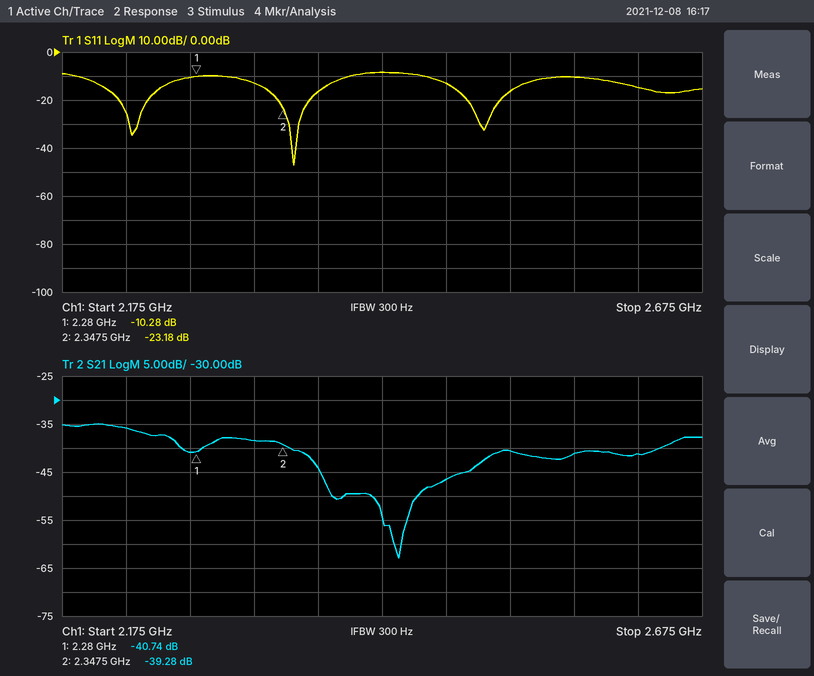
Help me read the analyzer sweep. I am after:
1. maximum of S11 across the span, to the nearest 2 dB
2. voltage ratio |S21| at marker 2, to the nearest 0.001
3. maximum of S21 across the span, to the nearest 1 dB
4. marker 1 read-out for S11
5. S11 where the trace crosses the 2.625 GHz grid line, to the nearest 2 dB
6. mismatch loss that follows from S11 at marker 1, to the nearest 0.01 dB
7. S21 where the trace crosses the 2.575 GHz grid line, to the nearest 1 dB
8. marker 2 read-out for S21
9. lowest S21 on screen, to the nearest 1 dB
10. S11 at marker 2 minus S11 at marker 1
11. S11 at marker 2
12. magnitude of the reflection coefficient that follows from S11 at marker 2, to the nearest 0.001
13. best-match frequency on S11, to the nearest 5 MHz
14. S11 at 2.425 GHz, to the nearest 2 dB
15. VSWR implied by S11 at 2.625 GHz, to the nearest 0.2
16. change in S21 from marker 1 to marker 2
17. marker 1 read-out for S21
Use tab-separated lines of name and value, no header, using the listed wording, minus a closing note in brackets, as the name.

maximum of S11 across the span, to the nearest 2 dB	-8 dB
voltage ratio |S21| at marker 2, to the nearest 0.001	0.011
maximum of S21 across the span, to the nearest 1 dB	-35 dB
marker 1 read-out for S11	-10.28 dB
S11 where the trace crosses the 2.625 GHz grid line, to the nearest 2 dB	-14 dB
mismatch loss that follows from S11 at marker 1, to the nearest 0.01 dB	0.43 dB
S21 where the trace crosses the 2.575 GHz grid line, to the nearest 1 dB	-41 dB
marker 2 read-out for S21	-39.28 dB
lowest S21 on screen, to the nearest 1 dB	-63 dB
S11 at marker 2 minus S11 at marker 1	-12.90 dB
S11 at marker 2	-23.18 dB
magnitude of the reflection coefficient that follows from S11 at marker 2, to the nearest 0.001	0.069
best-match frequency on S11, to the nearest 5 MHz	2.355 GHz
S11 at 2.425 GHz, to the nearest 2 dB	-8 dB
VSWR implied by S11 at 2.625 GHz, to the nearest 0.2	1.4
change in S21 from marker 1 to marker 2	1.46 dB
marker 1 read-out for S21	-40.74 dB
